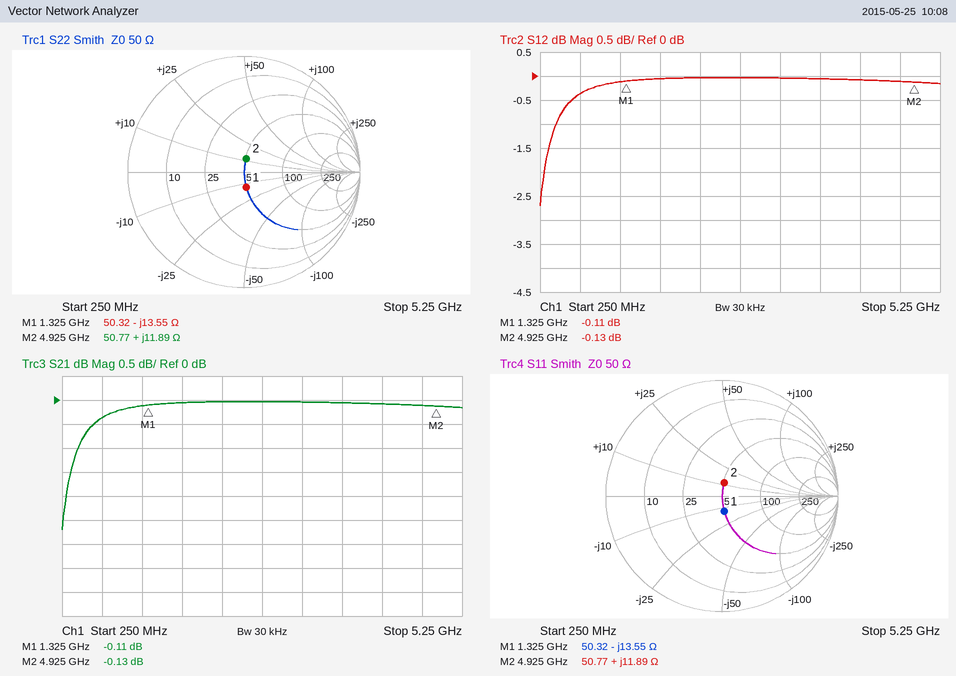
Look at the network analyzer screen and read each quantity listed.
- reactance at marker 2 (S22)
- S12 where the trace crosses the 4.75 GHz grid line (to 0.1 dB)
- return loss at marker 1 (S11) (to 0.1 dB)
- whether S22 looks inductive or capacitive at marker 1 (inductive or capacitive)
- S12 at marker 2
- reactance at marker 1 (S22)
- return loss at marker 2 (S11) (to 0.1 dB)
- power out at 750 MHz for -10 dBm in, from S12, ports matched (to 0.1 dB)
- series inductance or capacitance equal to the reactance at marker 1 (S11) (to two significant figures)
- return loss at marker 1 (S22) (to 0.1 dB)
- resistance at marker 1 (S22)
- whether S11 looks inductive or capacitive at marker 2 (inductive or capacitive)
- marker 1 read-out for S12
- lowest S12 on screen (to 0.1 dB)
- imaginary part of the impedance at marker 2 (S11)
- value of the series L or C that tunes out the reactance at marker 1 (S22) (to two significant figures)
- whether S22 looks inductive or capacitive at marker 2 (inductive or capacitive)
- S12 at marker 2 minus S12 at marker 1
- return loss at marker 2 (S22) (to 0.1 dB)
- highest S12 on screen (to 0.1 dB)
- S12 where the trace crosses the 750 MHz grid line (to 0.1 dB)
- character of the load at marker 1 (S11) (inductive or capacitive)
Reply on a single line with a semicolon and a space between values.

+11.89 Ω; -0.1 dB; 17.5 dB; capacitive; -0.13 dB; -13.55 Ω; 18.6 dB; -10.4 dBm; 8.9 pF; 17.5 dB; 50.32 Ω; inductive; -0.11 dB; -2.7 dB; +11.89 Ω; 1.6 nH; inductive; -0.02 dB; 18.6 dB; 0.0 dB; -0.4 dB; capacitive
